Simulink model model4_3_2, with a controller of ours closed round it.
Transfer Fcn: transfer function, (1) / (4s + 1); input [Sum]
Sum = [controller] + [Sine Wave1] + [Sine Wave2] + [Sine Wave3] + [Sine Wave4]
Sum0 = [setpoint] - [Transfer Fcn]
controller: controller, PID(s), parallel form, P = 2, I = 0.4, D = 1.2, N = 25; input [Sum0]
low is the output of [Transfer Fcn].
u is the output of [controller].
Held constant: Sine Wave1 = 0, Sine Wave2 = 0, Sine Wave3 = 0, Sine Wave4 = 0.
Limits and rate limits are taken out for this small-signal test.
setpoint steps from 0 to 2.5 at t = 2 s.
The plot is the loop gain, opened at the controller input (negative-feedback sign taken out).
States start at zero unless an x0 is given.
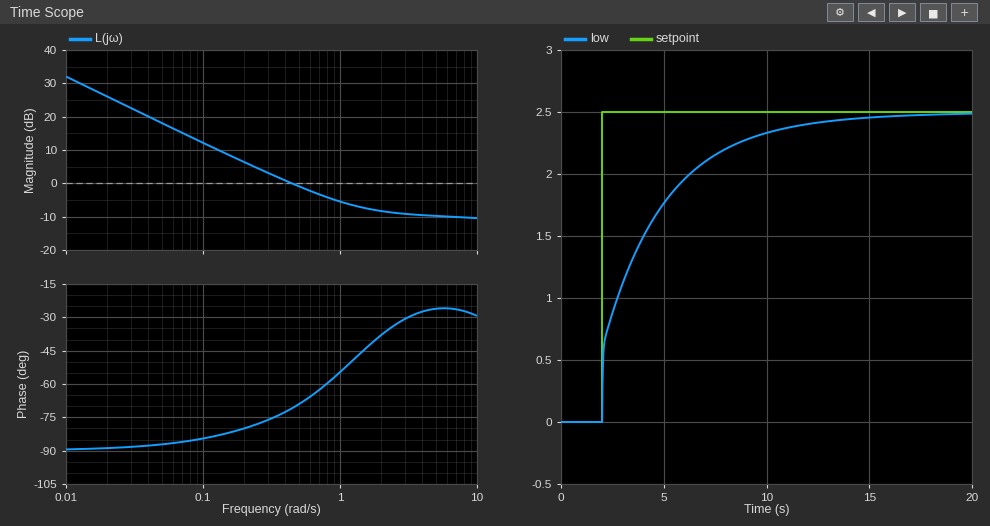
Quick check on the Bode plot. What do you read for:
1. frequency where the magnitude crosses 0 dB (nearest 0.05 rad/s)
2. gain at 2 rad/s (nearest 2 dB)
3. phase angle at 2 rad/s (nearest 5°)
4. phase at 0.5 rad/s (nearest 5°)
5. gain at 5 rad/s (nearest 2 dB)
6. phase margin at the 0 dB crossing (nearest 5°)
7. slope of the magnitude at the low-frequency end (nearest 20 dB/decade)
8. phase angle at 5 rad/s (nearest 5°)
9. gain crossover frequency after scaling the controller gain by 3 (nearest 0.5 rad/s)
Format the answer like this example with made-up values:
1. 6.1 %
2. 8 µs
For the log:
1. 0.45 rad/s
2. -8 dB
3. -40°
4. -70°
5. -10 dB
6. 110°
7. -20 dB/decade
8. -25°
9. 4.0 rad/s
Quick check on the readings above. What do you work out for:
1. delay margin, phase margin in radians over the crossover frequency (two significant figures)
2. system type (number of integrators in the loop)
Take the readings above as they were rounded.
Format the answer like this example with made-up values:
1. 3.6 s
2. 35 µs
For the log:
1. 4.3 s
2. 1
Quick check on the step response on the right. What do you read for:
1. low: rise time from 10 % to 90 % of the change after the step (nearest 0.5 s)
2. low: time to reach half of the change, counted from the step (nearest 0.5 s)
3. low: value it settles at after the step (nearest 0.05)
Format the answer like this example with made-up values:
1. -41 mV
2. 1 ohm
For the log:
1. 6.5 s
2. 1.5 s
3. 2.50
